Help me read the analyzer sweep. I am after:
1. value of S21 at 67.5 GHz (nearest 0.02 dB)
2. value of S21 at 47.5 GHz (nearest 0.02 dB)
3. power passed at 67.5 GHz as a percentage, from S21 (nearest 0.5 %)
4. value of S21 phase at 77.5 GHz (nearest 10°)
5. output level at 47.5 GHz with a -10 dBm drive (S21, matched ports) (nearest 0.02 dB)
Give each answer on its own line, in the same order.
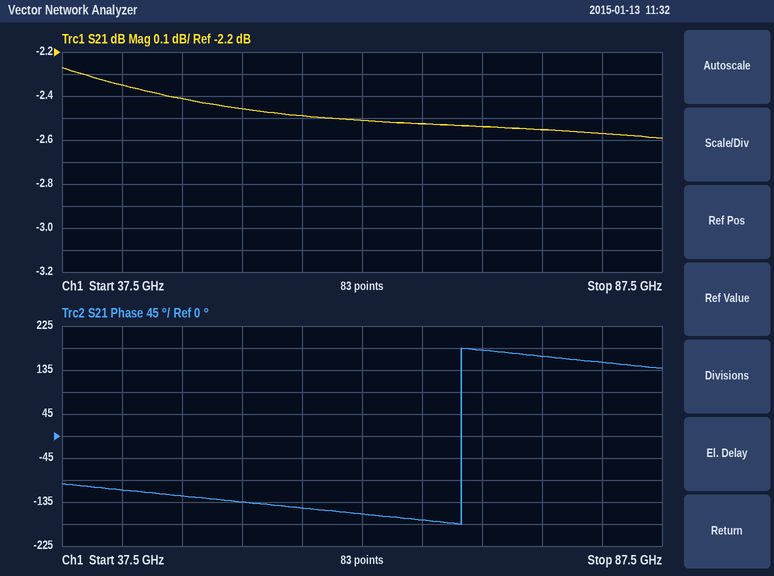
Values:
-2.52 dB
-2.42 dB
56.0 %
160°
-12.42 dBm
